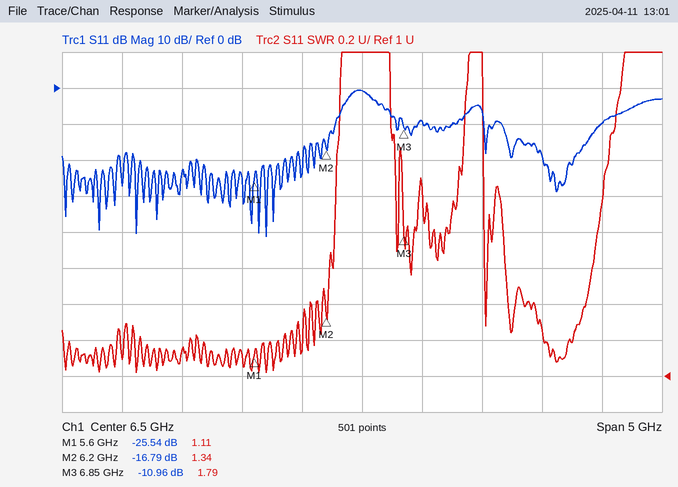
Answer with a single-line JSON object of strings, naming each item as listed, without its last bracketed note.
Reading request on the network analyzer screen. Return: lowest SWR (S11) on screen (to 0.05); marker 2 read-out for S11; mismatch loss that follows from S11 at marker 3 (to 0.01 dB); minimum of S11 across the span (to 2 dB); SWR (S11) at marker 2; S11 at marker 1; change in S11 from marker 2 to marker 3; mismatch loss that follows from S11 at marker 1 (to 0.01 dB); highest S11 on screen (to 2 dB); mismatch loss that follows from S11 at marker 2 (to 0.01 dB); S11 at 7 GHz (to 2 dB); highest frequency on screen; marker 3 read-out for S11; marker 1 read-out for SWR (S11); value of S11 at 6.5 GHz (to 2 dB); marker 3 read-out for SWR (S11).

{"lowest SWR (S11) on screen": "1.00", "marker 2 read-out for S11": "-16.79 dB", "mismatch loss that follows from S11 at marker 3": "0.36 dB", "minimum of S11 across the span": "-42 dB", "SWR (S11) at marker 2": "1.34", "S11 at marker 1": "-25.54 dB", "change in S11 from marker 2 to marker 3": "5.83 dB", "mismatch loss that follows from S11 at marker 1": "0.01 dB", "highest S11 on screen": "0 dB", "mismatch loss that follows from S11 at marker 2": "0.09 dB", "S11 at 7 GHz": "-10 dB", "highest frequency on screen": "9 GHz", "marker 3 read-out for S11": "-10.96 dB", "marker 1 read-out for SWR": "1.11", "value of S11 at 6.5 GHz": "0 dB", "marker 3 read-out for SWR": "1.79"}
